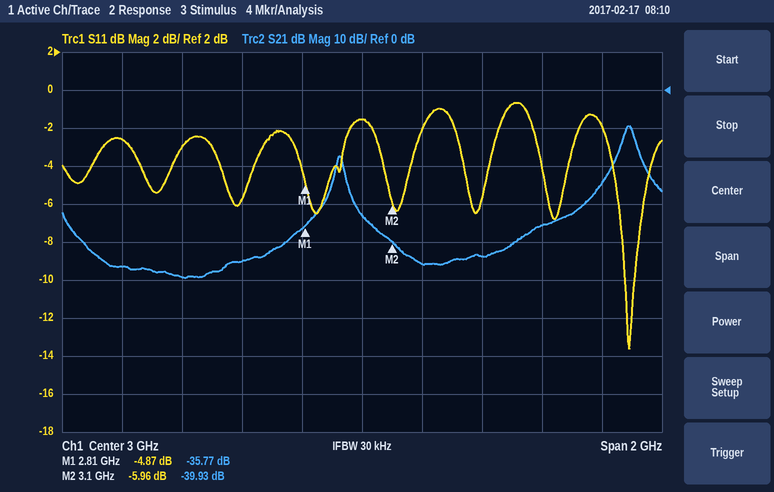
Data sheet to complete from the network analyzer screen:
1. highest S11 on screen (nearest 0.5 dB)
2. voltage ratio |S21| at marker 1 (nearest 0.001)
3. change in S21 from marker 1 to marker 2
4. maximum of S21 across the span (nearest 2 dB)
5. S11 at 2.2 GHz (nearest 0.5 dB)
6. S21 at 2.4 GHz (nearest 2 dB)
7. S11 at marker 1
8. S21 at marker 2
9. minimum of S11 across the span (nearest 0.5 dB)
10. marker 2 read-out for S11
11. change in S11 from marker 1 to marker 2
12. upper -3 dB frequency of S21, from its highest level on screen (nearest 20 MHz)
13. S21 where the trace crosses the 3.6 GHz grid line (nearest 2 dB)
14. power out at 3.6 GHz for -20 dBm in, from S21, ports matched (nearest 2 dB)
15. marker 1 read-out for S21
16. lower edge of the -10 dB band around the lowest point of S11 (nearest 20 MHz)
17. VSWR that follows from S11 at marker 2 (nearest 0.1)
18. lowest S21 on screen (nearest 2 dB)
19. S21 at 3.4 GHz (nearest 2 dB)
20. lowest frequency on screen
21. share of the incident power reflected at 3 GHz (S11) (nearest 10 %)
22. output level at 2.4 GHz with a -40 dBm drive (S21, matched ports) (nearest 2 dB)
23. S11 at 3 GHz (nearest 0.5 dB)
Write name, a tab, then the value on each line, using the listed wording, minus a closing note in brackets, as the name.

highest S11 on screen	-0.5 dB
voltage ratio |S21| at marker 1	0.016
change in S21 from marker 1 to marker 2	-4.16 dB
maximum of S21 across the span	-10 dB
S11 at 2.2 GHz	-2.5 dB
S21 at 2.4 GHz	-50 dB
S11 at marker 1	-4.87 dB
S21 at marker 2	-39.93 dB
minimum of S11 across the span	-13.5 dB
marker 2 read-out for S11	-5.96 dB
change in S11 from marker 1 to marker 2	-1.09 dB
upper -3 dB frequency of S21, from its highest level on screen	3.90 GHz
S21 where the trace crosses the 3.6 GHz grid line	-36 dB
power out at 3.6 GHz for -20 dBm in, from S21, ports matched	-56 dBm
marker 1 read-out for S21	-35.77 dB
lower edge of the -10 dB band around the lowest point of S11	3.88 GHz
VSWR that follows from S11 at marker 2	3.0
lowest S21 on screen	-50 dB
S21 at 3.4 GHz	-44 dB
lowest frequency on screen	2 GHz
share of the incident power reflected at 3 GHz (S11)	70 %
output level at 2.4 GHz with a -40 dBm drive (S21, matched ports)	-90 dBm
S11 at 3 GHz	-1.5 dB
